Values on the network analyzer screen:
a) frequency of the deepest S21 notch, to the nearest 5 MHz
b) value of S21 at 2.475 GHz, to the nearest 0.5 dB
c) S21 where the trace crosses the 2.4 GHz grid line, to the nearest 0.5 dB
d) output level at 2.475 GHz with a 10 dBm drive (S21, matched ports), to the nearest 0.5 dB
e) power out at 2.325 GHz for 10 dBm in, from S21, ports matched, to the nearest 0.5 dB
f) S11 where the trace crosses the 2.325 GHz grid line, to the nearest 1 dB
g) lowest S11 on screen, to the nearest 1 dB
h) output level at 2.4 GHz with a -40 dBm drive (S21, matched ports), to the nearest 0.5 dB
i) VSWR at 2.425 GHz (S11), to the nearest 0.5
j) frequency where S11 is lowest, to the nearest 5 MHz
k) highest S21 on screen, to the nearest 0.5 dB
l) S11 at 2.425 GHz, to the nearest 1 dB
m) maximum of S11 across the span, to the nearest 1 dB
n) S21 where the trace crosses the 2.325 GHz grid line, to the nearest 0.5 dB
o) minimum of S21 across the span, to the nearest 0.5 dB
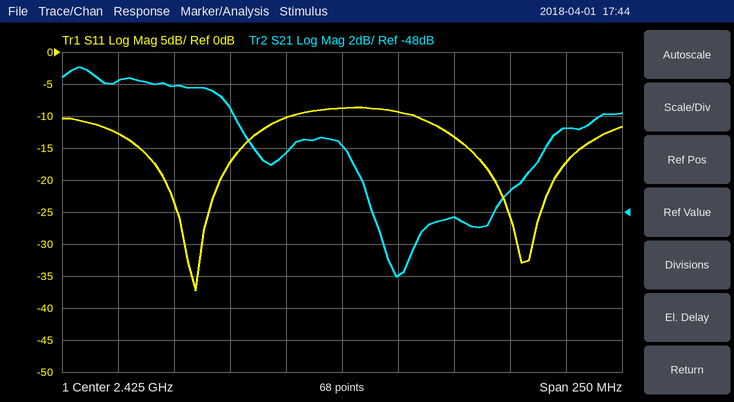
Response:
2.450 GHz
-48.5 dB
-44.5 dB
-38.5 dBm
-30.0 dBm
-13 dB
-37 dB
-84.5 dBm
2.0
2.360 GHz
-39.0 dB
-9 dB
-9 dB
-40.0 dB
-52.0 dB
